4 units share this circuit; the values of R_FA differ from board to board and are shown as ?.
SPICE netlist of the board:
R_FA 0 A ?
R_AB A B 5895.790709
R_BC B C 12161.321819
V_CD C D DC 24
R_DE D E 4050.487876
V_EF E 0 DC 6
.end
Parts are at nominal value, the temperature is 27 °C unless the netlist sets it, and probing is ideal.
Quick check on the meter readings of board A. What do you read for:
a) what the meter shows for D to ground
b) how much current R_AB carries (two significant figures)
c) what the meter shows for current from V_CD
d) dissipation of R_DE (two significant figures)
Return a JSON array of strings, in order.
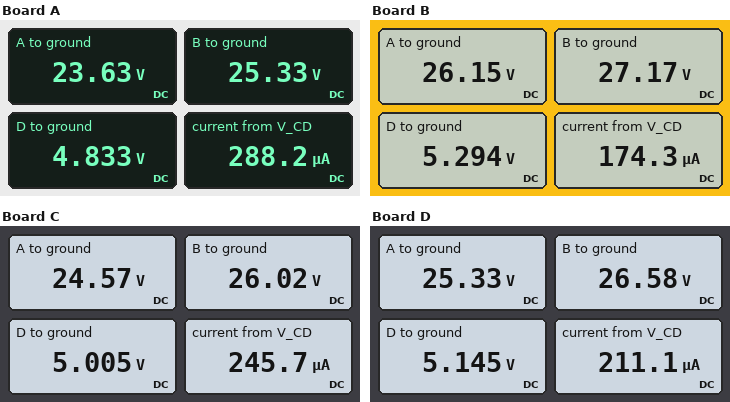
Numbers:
["4.833 V", "290 µA", "288.2 µA", "340 µW"]
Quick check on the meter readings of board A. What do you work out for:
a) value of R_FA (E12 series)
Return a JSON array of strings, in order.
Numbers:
["82 kΩ"]
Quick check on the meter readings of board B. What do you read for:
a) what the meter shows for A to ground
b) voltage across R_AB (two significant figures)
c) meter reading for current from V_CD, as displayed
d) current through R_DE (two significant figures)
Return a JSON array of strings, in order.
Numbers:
["26.15 V", "1.0 V", "174.3 µA", "170 µA"]
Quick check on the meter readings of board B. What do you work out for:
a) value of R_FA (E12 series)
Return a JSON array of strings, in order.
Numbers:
["150 kΩ"]
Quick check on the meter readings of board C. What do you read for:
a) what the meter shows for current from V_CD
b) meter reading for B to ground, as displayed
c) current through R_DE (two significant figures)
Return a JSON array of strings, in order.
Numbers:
["245.7 µA", "26.02 V", "250 µA"]
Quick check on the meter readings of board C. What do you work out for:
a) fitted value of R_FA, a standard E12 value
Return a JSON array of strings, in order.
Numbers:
["100 kΩ"]
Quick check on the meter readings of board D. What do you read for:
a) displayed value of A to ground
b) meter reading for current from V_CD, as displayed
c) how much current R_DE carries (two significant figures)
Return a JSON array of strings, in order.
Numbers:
["25.33 V", "211.1 µA", "210 µA"]
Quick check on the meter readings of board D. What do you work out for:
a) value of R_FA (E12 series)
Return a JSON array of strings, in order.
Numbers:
["120 kΩ"]
